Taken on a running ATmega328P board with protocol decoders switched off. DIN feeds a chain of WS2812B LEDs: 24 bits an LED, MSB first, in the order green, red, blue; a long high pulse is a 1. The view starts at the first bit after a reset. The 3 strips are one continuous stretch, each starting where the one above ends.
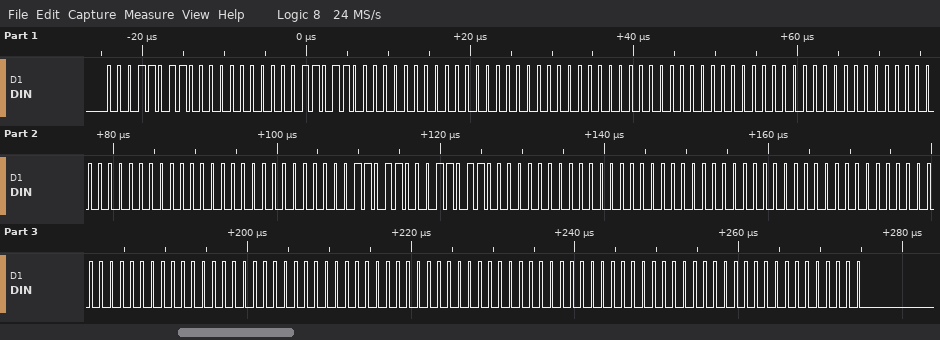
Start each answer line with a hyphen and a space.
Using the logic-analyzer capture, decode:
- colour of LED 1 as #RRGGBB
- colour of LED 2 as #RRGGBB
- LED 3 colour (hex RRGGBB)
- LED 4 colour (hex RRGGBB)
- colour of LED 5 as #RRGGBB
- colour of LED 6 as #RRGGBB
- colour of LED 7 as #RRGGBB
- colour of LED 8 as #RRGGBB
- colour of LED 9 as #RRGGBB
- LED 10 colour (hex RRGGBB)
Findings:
- #001B1B
- #000000
- #000000
- #000000
- #1B001B
- #000000
- #000000
- #000000
- #000000
- #000000
